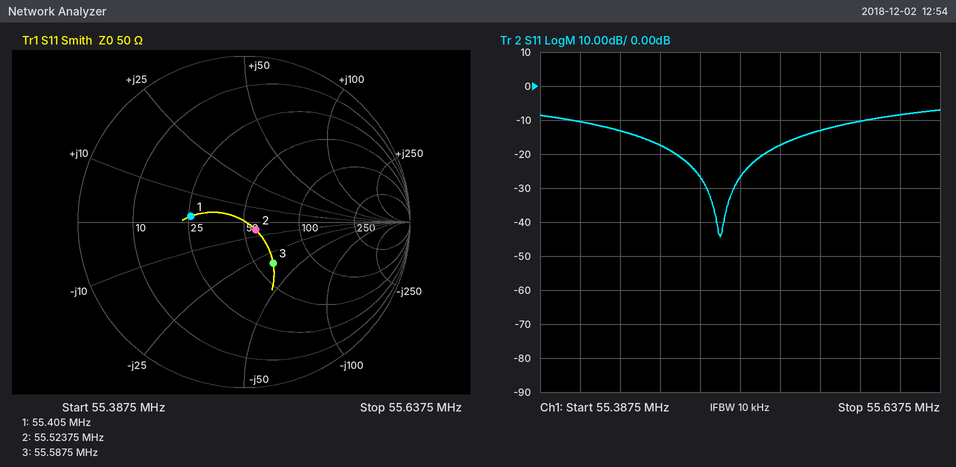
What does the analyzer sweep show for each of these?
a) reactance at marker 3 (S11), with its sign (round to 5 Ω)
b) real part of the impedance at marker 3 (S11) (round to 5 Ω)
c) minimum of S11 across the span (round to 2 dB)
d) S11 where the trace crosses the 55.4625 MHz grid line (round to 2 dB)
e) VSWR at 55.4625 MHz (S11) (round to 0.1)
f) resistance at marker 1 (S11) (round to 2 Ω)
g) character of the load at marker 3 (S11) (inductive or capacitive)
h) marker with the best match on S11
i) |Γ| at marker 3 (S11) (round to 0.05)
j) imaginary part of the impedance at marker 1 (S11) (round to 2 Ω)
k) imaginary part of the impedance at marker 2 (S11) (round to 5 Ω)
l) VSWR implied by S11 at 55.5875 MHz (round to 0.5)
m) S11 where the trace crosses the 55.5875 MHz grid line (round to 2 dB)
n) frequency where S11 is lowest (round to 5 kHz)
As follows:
-35 Ω
60 Ω
-44 dB
-18 dB
1.3
26 Ω
capacitive
marker 2
0.30
+2 Ω
-5 Ω
2.0
-10 dB
55.500 MHz
